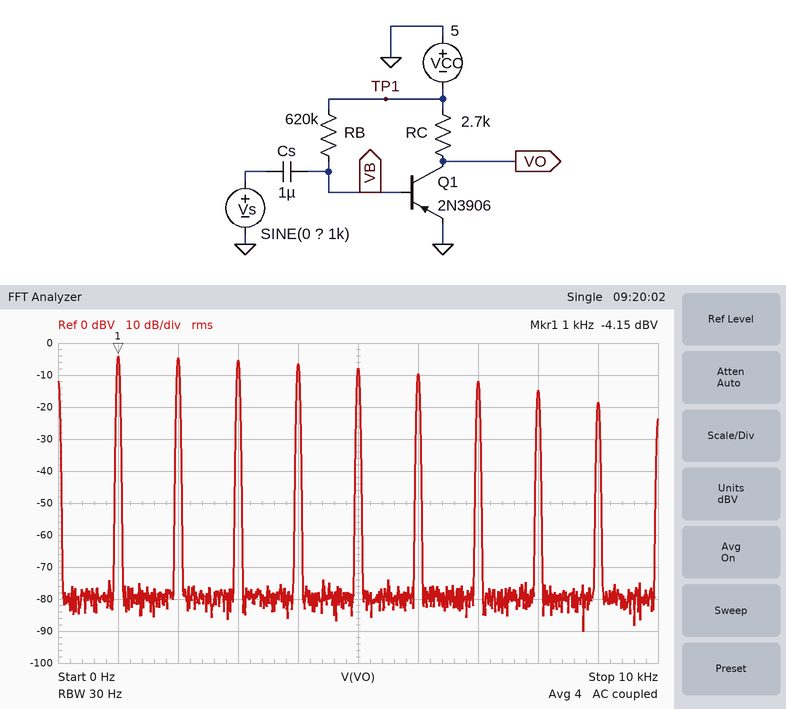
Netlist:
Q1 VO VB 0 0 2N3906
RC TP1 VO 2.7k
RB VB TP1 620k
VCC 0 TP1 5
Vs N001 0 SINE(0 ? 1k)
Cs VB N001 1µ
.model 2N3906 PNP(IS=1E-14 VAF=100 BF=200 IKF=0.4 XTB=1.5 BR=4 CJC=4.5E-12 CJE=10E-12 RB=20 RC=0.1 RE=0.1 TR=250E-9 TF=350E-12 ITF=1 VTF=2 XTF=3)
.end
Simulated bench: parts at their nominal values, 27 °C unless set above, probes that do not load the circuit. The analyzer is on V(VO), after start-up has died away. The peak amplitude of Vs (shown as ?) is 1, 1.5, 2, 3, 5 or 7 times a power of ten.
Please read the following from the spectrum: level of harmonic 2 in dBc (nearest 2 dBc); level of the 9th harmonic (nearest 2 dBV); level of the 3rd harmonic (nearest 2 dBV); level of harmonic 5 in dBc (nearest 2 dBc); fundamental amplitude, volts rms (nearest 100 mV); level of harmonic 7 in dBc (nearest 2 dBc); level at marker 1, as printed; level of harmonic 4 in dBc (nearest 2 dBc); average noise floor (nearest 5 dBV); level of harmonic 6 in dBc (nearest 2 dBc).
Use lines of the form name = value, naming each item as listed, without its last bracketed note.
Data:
level of harmonic 2 in dBc = 0 dBc
level of the 9th harmonic = -18 dBV
level of the 3rd harmonic = -6 dBV
level of harmonic 5 in dBc = -4 dBc
fundamental amplitude, volts rms = 600 mV
level of harmonic 7 in dBc = -8 dBc
level at marker 1, as printed = -4.15 dBV
level of harmonic 4 in dBc = -2 dBc
average noise floor = -80 dBV
level of harmonic 6 in dBc = -6 dBc
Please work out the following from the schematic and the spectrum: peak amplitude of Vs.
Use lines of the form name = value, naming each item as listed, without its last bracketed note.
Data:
peak amplitude of Vs = 1 V
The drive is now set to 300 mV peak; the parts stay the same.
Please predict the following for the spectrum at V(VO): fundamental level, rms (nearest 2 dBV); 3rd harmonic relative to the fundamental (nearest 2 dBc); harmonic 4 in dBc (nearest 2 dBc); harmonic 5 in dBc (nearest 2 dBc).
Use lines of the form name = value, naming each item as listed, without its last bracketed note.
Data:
fundamental level, rms = 0 dBV
3rd harmonic relative to the fundamental = -4 dBc
harmonic 4 in dBc = -8 dBc
harmonic 5 in dBc = -12 dBc
